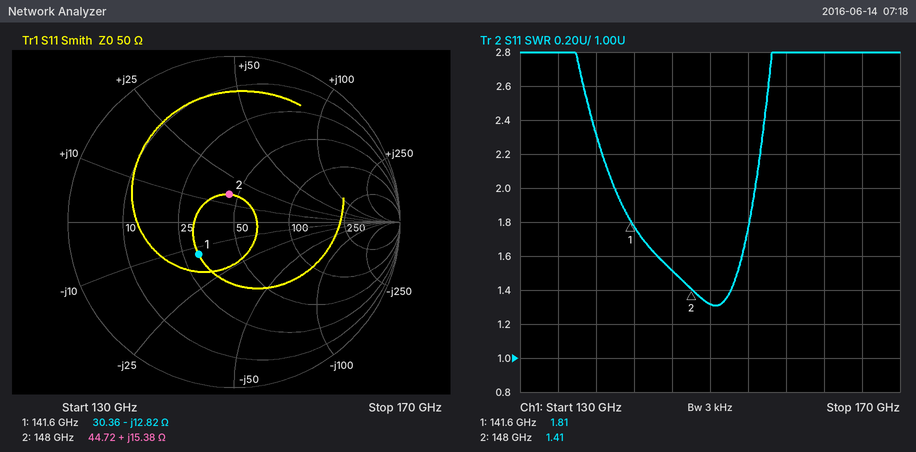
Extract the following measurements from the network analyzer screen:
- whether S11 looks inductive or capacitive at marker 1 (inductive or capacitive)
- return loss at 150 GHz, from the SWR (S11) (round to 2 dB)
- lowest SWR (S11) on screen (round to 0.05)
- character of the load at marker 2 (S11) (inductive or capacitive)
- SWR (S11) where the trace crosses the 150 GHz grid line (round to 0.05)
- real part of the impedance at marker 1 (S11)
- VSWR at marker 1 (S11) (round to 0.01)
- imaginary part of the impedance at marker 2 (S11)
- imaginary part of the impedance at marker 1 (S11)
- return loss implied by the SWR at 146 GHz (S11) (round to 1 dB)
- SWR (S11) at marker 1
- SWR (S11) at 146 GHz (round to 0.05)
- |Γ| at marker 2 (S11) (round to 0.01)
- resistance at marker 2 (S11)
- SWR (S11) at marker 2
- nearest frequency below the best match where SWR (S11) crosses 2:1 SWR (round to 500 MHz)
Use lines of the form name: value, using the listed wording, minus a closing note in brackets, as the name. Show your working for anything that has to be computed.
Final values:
whether S11 looks inductive or capacitive at marker 1: capacitive
return loss at 150 GHz, from the SWR (S11): −20 log10((1.3 − 1)/(1.3 + 1)) ≈ 18 dB
lowest SWR (S11) on screen: 1.30
character of the load at marker 2 (S11): inductive
SWR (S11) where the trace crosses the 150 GHz grid line: 1.30
real part of the impedance at marker 1: 30.36 Ω
VSWR at marker 1 (S11): 1.81
imaginary part of the impedance at marker 2: +15.38 Ω
imaginary part of the impedance at marker 1: -12.82 Ω
return loss implied by the SWR at 146 GHz (S11): −20 log10((1.5 − 1)/(1.5 + 1)) ≈ 14 dB
SWR (S11) at marker 1: 1.81
SWR (S11) at 146 GHz: 1.50
|Γ| at marker 2 (S11): 0.17
resistance at marker 2: 44.72 Ω
SWR (S11) at marker 2: 1.41
nearest frequency below the best match where SWR (S11) crosses 2:1 SWR: 140.0 GHz
